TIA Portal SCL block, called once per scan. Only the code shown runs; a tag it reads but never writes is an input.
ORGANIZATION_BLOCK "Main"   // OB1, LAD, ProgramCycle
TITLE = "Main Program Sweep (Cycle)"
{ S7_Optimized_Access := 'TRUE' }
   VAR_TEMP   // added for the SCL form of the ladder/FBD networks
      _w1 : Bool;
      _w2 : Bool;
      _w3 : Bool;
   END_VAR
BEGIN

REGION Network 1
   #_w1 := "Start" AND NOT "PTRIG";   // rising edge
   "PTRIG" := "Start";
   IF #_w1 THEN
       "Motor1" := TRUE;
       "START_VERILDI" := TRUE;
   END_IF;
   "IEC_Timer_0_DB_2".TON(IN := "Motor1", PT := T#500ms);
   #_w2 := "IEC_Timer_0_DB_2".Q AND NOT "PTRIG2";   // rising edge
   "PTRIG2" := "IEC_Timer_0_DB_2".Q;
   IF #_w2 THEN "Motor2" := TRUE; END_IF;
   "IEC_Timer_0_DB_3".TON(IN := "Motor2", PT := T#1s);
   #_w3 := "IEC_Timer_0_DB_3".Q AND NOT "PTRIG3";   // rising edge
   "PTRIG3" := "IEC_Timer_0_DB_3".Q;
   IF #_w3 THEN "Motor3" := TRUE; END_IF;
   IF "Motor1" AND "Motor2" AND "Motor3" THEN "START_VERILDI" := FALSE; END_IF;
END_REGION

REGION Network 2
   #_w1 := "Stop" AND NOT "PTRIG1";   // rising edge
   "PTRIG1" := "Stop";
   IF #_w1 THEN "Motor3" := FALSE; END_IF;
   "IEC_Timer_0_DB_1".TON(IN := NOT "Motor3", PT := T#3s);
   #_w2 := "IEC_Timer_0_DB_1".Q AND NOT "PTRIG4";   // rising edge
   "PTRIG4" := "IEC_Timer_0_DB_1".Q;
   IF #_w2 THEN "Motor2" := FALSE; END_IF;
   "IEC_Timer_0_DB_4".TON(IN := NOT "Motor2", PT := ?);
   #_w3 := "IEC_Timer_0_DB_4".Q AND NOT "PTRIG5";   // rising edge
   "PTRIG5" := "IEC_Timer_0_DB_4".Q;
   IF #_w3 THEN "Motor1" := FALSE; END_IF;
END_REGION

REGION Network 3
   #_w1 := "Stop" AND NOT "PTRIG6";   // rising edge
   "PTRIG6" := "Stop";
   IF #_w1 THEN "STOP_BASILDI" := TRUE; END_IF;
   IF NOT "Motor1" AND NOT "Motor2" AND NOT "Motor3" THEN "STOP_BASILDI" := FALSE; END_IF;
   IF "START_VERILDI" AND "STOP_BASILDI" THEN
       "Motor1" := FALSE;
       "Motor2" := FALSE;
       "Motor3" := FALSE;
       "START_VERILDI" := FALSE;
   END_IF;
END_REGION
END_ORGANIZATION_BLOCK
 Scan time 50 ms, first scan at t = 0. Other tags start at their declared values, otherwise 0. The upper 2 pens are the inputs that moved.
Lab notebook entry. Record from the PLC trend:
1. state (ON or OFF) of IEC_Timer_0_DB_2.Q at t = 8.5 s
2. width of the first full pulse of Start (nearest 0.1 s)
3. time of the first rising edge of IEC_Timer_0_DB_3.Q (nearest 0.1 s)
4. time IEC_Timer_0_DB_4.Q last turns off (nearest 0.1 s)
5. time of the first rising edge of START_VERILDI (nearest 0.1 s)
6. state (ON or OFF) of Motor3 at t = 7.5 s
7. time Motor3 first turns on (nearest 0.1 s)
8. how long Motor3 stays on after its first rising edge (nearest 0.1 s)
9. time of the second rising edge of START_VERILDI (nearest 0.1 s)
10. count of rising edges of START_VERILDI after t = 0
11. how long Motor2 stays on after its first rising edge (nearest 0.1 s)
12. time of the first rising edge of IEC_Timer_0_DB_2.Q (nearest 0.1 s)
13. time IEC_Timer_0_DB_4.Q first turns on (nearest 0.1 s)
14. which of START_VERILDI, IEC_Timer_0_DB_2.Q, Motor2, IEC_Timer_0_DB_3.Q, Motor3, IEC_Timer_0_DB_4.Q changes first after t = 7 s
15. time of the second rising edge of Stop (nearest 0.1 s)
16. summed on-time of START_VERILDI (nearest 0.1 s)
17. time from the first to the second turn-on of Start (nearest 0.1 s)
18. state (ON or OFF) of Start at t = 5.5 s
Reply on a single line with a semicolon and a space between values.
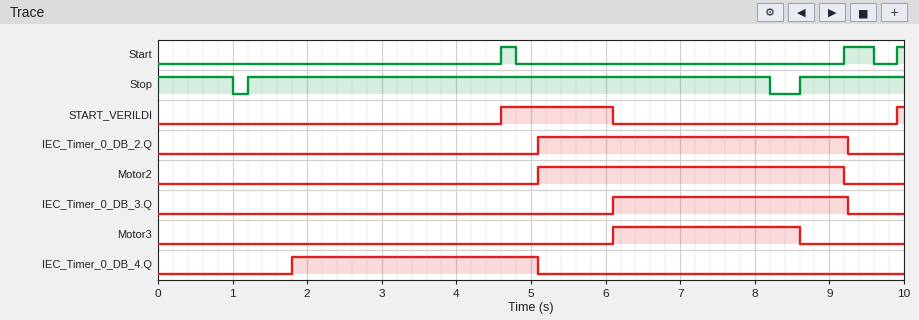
ON; 0.2 s; 6.1 s; 5.1 s; 4.6 s; ON; 6.1 s; 2.5 s; 9.9 s; 2; 4.1 s; 5.1 s; 1.8 s; Motor3; 8.6 s; 1.6 s; 4.6 s; OFF
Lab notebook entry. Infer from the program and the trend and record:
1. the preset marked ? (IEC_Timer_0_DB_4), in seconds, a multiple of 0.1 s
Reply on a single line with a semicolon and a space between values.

1.8 s
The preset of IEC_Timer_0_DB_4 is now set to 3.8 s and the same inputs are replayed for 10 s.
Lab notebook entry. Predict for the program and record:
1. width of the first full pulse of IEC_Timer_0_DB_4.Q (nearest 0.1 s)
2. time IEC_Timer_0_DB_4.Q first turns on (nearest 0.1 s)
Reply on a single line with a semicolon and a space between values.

1.3 s; 3.8 s
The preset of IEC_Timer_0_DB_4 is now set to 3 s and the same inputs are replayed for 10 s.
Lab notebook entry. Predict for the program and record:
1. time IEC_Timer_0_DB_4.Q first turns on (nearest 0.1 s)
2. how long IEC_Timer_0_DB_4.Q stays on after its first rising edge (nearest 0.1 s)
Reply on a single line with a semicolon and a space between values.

3.0 s; 2.1 s
